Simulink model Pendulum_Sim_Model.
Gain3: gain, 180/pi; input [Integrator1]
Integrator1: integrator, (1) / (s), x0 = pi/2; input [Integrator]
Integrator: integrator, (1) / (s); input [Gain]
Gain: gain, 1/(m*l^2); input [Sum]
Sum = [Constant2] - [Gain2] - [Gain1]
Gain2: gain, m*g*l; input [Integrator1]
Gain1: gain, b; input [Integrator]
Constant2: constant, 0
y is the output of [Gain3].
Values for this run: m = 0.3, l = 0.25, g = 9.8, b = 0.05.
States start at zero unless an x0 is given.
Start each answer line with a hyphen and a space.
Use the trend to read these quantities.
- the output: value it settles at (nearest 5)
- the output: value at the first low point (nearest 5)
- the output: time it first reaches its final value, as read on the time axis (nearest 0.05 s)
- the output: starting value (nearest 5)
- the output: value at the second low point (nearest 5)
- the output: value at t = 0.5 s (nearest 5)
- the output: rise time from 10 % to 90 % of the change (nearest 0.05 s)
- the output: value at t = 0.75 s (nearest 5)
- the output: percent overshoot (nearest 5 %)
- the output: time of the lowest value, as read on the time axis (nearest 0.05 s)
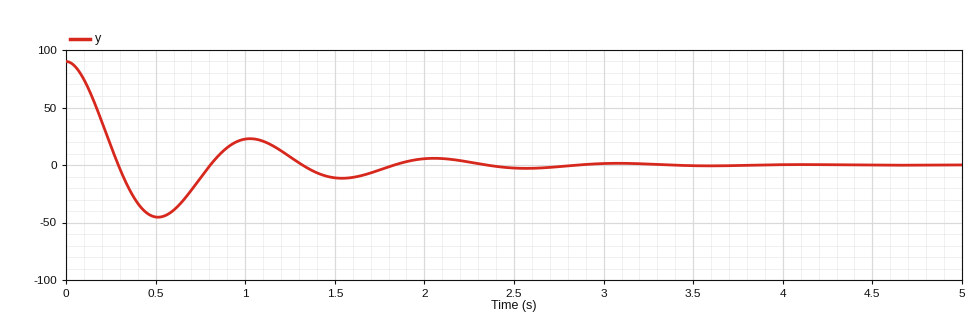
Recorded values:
- 0
- -45
- 0.30 s
- 90
- -10
- -45
- 0.20 s
- -10
- 50 %
- 0.50 s
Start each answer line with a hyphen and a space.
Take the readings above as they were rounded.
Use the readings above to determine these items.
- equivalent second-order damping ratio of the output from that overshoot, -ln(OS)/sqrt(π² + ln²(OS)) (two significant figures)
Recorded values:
- 0.22
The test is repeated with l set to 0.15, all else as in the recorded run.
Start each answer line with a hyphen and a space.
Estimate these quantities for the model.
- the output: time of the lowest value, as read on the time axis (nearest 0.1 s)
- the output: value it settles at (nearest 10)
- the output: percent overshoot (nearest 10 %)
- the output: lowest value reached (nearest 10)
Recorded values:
- 0.4 s
- 0
- 20 %
- -20
